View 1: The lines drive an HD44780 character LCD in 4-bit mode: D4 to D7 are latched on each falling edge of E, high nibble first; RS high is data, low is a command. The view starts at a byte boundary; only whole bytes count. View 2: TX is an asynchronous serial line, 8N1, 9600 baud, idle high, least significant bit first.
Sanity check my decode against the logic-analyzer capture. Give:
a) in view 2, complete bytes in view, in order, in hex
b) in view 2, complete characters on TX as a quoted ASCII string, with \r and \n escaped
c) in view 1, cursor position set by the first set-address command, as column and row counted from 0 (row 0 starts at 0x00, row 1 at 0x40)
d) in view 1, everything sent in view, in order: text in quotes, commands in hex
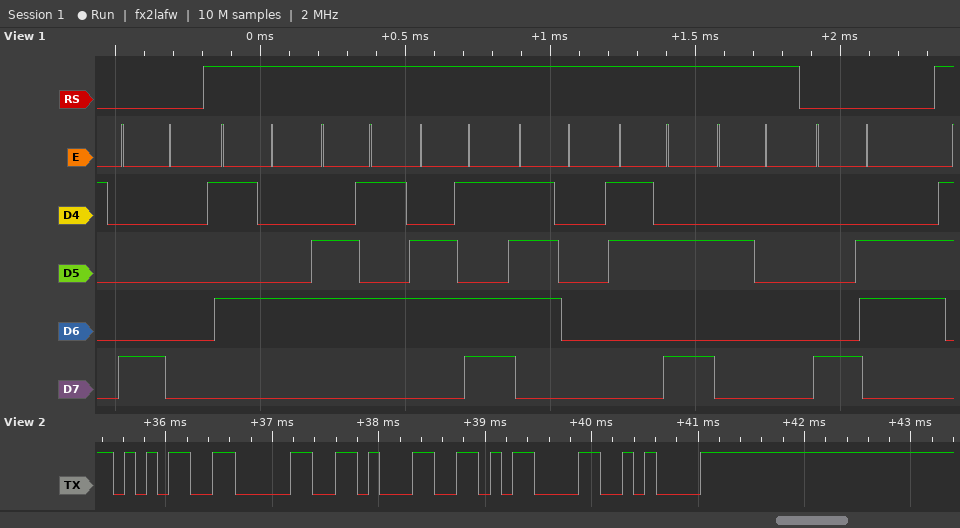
0x35 0x30 0x31 0x0D 0x0A
"501\r\n"
column 0, row 0
0x80 "Temp: " 0x86
